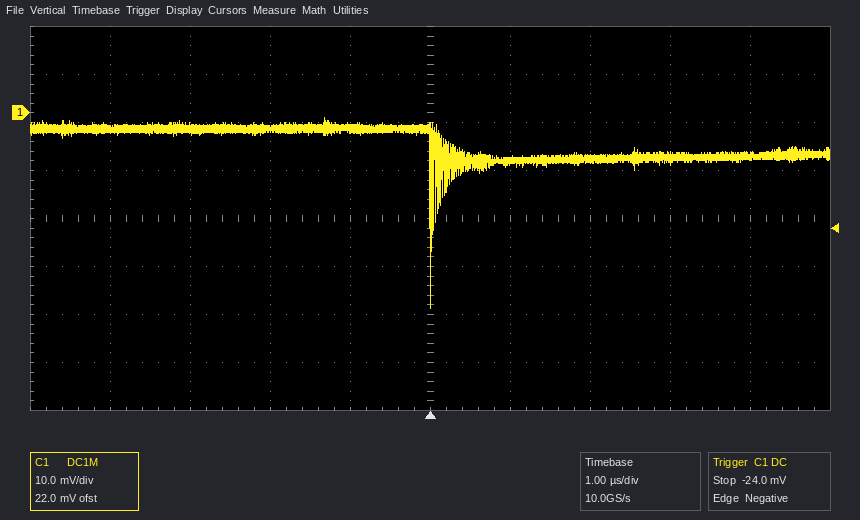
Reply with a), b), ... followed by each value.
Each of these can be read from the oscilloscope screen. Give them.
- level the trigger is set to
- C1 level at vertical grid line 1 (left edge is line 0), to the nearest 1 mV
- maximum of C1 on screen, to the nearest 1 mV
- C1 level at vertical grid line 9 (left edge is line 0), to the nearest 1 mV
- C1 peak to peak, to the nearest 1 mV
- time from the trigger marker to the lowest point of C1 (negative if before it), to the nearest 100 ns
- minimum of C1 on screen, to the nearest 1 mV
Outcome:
a) -24.0 mV
b) -3 mV
c) -1 mV
d) -9 mV
e) 40 mV
f) 0.0 µs
g) -41 mV
